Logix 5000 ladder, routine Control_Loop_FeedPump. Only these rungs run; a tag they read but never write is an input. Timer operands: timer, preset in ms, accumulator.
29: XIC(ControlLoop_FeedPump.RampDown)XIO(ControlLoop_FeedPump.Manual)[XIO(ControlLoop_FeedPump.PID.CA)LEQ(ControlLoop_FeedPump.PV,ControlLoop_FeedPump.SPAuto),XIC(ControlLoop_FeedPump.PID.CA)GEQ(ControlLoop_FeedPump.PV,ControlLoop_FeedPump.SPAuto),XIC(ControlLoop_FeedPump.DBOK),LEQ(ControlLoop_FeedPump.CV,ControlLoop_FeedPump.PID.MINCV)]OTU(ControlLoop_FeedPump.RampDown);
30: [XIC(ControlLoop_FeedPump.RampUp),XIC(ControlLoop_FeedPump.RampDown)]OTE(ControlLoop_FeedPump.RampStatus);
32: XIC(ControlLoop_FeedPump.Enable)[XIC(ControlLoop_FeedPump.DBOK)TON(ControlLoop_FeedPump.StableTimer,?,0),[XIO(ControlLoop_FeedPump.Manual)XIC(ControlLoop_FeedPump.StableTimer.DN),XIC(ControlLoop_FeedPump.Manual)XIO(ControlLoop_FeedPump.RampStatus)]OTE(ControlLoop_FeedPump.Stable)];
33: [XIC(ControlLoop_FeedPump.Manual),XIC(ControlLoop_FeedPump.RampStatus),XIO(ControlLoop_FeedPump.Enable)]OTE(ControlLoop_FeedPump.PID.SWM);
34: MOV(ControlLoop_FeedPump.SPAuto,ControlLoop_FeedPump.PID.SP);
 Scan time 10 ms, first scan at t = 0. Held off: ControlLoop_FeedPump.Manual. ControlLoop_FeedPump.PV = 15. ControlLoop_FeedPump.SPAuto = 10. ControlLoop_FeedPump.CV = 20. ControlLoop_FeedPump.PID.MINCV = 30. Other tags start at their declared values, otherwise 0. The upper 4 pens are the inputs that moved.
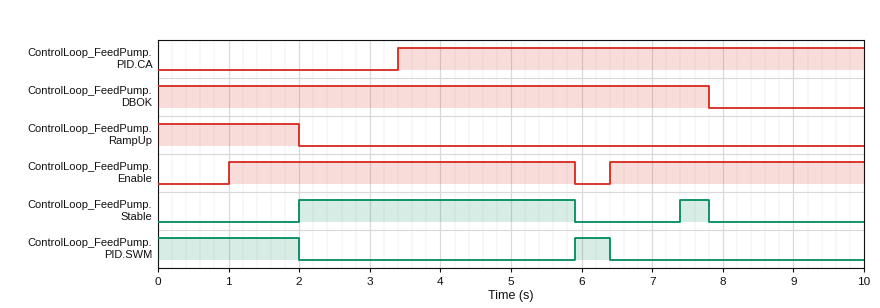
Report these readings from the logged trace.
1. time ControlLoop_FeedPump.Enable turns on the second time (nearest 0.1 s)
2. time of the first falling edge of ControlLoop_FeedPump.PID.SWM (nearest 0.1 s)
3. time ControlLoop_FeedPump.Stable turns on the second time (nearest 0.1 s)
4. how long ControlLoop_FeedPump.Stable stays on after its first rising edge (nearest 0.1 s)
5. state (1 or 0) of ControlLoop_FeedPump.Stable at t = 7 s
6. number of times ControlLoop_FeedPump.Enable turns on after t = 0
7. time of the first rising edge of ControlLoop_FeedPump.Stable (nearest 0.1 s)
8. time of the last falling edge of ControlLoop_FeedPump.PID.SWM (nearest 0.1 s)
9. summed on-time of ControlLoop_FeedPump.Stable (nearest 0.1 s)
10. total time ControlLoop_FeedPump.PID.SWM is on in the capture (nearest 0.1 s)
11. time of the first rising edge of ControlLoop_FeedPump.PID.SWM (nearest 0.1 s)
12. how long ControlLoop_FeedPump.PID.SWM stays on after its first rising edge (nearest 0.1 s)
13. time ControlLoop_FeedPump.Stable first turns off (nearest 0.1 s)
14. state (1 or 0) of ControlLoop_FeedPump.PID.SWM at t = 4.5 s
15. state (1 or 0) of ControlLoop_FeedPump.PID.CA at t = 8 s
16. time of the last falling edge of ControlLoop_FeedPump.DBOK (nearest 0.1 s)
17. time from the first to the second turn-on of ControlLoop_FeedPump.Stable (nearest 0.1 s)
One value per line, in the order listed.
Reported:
6.4 s
2.0 s
7.4 s
3.9 s
0
2
2.0 s
6.4 s
4.3 s
2.5 s
5.9 s
0.5 s
5.9 s
0
1
7.8 s
5.4 s
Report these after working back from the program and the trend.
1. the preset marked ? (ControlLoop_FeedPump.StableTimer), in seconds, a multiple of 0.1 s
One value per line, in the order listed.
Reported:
1.0 s
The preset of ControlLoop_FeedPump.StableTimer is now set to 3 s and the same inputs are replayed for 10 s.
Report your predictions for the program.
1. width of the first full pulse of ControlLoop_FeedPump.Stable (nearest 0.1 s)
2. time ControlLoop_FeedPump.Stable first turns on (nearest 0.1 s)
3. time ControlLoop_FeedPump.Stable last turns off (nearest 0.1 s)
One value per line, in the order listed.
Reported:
1.9 s
4.0 s
5.9 s
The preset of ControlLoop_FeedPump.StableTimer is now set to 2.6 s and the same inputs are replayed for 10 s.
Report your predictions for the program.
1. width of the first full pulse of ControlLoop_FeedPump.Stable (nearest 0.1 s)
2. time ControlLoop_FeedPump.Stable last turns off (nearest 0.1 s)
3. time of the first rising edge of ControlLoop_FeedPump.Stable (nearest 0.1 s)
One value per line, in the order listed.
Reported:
2.3 s
5.9 s
3.6 s
